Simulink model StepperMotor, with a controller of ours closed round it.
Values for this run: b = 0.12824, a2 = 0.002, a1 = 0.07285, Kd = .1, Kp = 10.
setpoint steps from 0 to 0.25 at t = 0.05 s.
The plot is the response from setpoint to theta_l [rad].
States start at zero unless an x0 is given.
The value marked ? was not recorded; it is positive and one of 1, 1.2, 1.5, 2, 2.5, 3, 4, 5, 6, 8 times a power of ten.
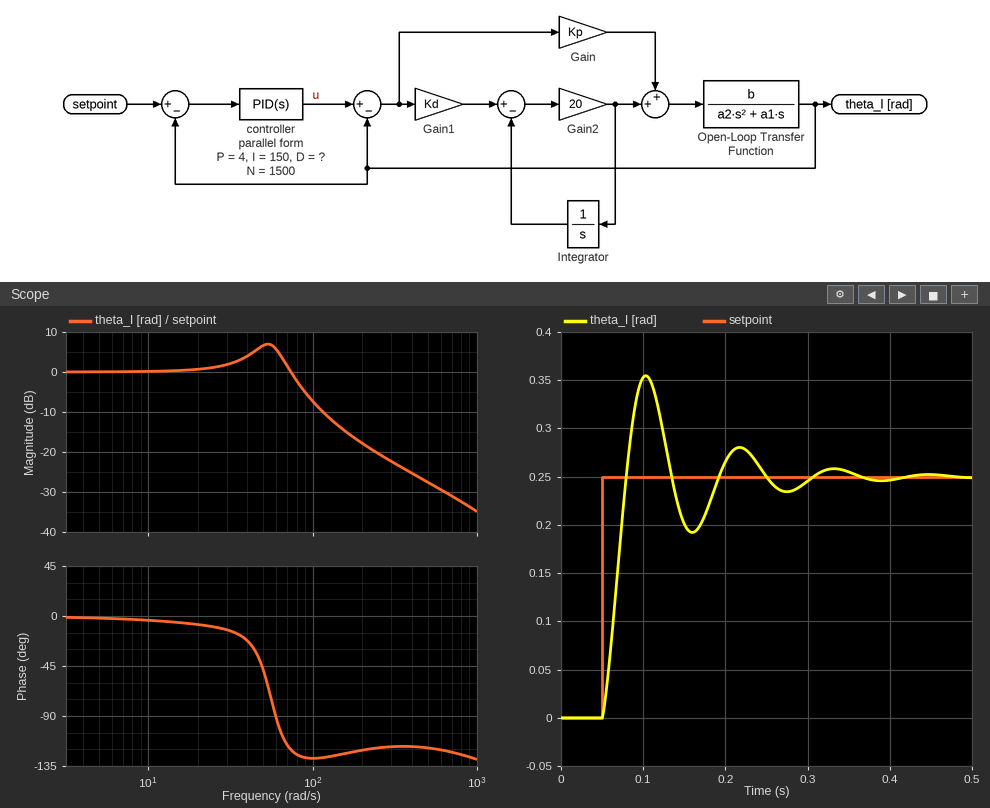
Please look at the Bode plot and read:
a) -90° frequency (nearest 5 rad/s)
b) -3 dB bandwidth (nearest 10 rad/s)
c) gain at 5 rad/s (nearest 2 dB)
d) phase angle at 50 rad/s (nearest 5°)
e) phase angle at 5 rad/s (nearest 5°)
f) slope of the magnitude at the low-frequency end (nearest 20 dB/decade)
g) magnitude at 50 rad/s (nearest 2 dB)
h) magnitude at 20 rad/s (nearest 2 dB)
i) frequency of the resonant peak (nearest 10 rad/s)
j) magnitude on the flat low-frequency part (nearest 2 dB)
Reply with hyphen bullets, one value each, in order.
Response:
- 60 rad/s
- 80 rad/s
- 0 dB
- -50°
- 0°
- 0 dB/decade
- 6 dB
- 0 dB
- 50 rad/s
- 0 dB
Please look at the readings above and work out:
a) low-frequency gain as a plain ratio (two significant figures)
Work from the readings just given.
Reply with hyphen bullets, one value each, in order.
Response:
- 1.0
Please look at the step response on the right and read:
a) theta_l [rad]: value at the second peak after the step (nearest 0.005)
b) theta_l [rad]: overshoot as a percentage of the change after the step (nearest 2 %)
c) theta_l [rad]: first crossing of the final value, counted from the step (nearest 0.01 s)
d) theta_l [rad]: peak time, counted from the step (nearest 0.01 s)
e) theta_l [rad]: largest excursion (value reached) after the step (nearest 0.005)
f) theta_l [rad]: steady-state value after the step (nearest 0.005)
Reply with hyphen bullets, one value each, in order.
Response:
- 0.280
- 42 %
- 0.03 s
- 0.05 s
- 0.355
- 0.250
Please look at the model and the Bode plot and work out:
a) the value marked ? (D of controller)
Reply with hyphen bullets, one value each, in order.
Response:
- 0.025
